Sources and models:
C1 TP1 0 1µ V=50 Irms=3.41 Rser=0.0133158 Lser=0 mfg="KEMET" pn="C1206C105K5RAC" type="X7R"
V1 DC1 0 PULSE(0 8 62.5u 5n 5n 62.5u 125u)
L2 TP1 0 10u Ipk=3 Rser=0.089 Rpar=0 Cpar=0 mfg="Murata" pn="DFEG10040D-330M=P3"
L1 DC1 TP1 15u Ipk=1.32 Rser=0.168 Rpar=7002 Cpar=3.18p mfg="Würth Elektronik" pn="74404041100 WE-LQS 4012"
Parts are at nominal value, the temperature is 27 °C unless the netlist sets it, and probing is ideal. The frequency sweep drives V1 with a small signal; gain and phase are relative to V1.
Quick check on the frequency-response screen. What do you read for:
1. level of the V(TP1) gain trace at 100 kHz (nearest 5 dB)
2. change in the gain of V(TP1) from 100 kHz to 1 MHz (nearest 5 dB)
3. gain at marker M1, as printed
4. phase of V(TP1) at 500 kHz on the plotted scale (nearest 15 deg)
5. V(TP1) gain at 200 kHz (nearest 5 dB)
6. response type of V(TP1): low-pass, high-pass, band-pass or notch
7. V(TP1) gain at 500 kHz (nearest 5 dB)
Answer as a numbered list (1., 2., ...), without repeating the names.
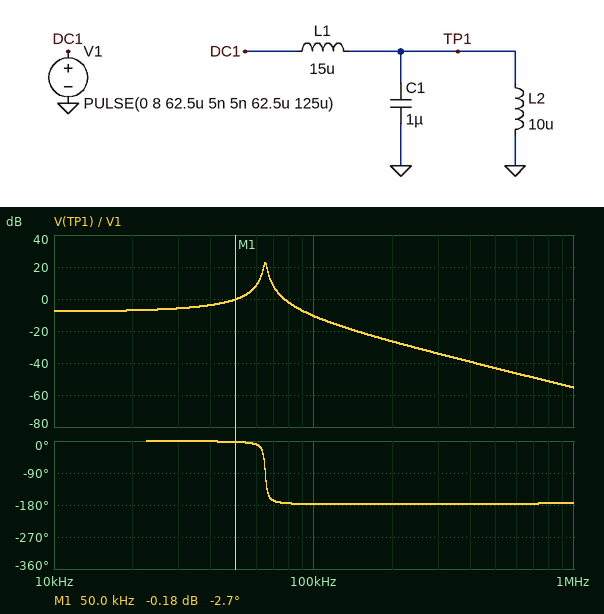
1. -10 dB
2. -45 dB
3. -0.18 dB
4. -180 deg
5. -25 dB
6. low-pass
7. -45 dB
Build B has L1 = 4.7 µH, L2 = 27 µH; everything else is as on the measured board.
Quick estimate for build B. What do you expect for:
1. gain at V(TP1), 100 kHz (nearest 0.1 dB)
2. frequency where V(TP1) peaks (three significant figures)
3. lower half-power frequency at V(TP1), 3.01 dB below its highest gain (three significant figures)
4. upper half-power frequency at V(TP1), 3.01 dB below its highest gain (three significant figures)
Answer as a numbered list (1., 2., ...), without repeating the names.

1. 3.2 dB
2. 79.4 kHz
3. 76.6 kHz
4. 82.1 kHz
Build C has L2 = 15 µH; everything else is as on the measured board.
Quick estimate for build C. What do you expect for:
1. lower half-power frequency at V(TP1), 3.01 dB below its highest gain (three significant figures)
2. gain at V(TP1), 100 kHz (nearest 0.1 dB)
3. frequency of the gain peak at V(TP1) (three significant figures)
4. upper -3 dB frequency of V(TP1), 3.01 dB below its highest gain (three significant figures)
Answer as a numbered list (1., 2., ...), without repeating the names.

1. 57.3 kHz
2. -11.9 dB
3. 58.1 kHz
4. 58.9 kHz
